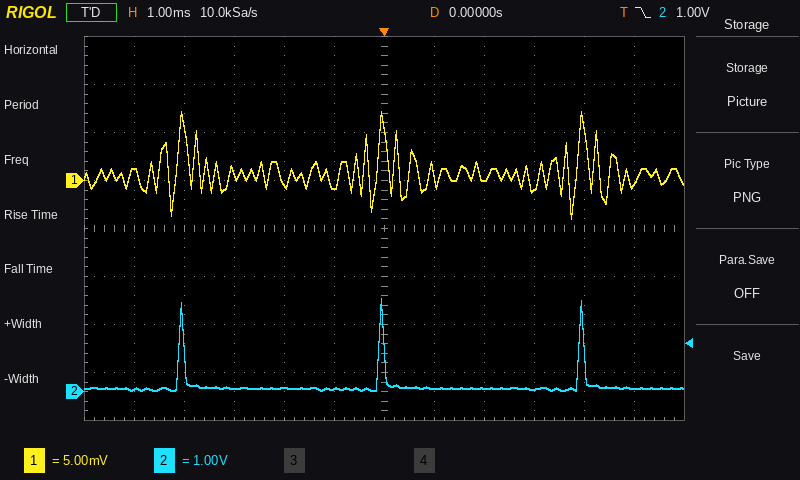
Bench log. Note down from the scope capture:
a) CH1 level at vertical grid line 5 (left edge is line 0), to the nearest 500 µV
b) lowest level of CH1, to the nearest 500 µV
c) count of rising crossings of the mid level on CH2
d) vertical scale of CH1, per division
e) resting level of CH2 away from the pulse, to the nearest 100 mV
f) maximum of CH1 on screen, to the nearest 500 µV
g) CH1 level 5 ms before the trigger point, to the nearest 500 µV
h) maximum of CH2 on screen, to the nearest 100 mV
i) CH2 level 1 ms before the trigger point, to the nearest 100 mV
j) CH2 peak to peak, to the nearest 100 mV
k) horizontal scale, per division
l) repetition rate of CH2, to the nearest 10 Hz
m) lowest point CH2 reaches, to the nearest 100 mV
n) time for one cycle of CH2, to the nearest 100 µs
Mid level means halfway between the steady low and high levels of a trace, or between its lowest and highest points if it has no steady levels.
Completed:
-500 µV
-4.0 mV
3
5 mV
100 mV
7.0 mV
1.0 mV
1.9 V
100 mV
1.9 V
1 ms
250 Hz
0.0 V
4.0 ms
